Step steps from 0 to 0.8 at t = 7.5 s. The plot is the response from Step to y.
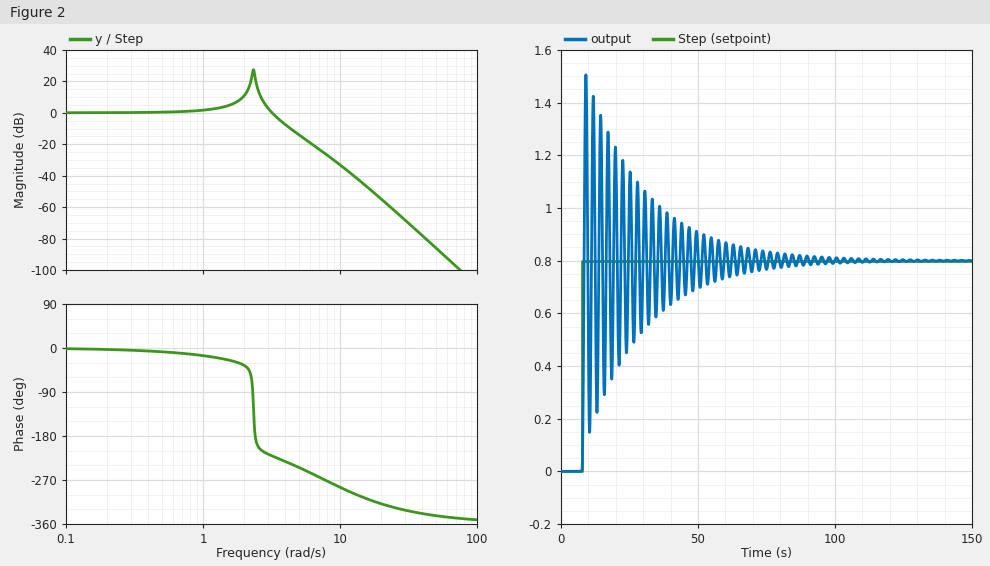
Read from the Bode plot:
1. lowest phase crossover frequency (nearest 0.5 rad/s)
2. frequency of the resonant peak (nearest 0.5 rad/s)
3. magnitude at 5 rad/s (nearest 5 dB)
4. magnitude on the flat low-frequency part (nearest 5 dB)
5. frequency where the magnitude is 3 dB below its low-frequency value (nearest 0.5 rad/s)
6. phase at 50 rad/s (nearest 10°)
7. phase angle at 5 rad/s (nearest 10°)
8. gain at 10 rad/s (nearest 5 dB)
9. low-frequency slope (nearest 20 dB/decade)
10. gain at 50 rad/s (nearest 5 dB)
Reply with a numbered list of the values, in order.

1. 2.5 rad/s
2. 2.5 rad/s
3. -15 dB
4. 0 dB
5. 3.5 rad/s
6. -340°
7. -240°
8. -35 dB
9. 0 dB/decade
10. -85 dB
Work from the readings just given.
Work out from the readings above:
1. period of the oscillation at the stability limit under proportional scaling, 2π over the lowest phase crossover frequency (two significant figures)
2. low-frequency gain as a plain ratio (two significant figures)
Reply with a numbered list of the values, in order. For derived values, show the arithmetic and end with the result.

1. 2π / 2.5 = 2.5 s
2. 10^(0 / 20) = 1.0
